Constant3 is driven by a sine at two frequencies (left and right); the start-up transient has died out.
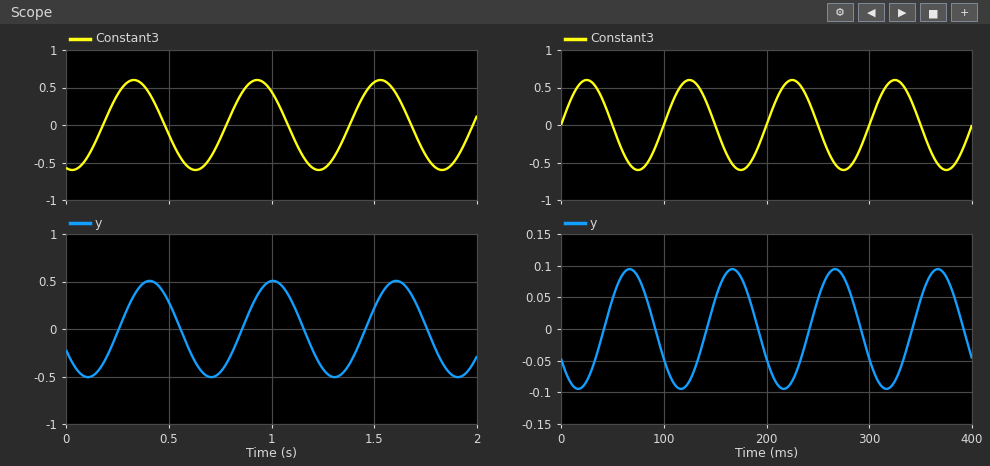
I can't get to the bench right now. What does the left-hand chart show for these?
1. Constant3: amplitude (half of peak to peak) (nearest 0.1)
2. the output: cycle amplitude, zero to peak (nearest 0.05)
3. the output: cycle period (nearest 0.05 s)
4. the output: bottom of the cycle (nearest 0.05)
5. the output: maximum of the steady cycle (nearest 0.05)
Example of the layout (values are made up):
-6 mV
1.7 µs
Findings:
0.6
0.50
0.60 s
-0.50
0.50
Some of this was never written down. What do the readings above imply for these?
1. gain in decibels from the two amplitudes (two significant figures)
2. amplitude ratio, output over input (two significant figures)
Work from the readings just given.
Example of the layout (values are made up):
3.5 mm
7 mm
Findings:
-1.6 dB
0.83
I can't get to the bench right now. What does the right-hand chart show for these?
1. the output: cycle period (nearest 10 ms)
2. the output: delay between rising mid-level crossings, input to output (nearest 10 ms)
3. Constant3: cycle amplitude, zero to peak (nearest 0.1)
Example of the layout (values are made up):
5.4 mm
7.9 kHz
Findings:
100 ms
40 ms
0.6
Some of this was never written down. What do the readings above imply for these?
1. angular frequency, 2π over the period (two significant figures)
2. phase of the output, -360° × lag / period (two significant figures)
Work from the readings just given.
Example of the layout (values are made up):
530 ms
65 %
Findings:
0.063 rad/ms
-140°
